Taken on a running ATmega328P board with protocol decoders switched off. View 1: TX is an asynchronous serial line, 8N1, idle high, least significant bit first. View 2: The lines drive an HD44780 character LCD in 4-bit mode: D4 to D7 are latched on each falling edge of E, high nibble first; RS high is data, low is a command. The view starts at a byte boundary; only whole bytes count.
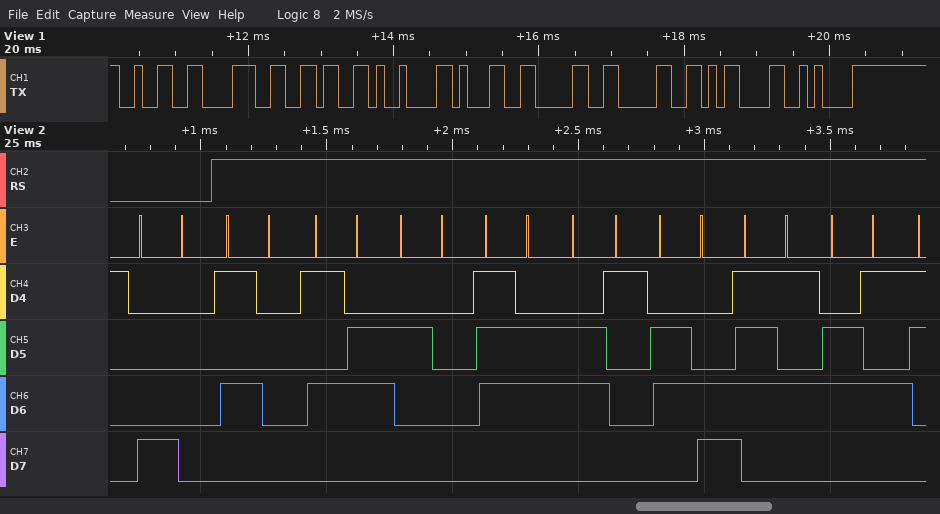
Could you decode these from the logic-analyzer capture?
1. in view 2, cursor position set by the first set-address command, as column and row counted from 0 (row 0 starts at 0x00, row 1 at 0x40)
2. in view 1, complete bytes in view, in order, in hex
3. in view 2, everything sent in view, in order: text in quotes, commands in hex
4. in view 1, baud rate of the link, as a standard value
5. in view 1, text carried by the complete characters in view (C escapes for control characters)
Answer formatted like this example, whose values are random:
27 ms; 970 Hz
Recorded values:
column 0, row 0; 32 38 36 09 31 30 30 0D 0A; 0x80 "PV value"; 9600 baud; "286\t100\r\n"
